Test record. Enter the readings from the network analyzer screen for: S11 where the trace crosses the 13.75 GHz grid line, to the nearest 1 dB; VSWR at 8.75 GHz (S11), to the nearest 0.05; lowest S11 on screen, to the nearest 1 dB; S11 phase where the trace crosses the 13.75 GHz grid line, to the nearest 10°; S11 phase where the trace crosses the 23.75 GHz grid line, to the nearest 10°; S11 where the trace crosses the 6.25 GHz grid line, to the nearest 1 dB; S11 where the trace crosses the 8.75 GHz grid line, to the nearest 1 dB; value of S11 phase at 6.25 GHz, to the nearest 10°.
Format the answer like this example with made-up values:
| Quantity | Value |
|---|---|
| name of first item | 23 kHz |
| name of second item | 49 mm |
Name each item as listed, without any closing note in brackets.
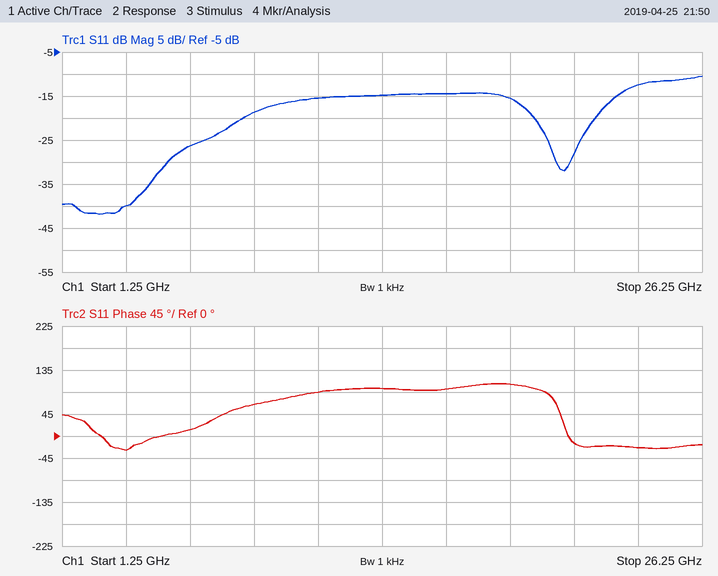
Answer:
| Quantity | Value |
|---|---|
| S11 where the trace crosses the 13.75 GHz grid line, to the nearest 1 dB | -15 dB |
| VSWR at 8.75 GHz (S11), to the nearest 0.05 | 1.25 |
| lowest S11 on screen, to the nearest 1 dB | -42 dB |
| S11 phase where the trace crosses the 13.75 GHz grid line, to the nearest 10° | 100° |
| S11 phase where the trace crosses the 23.75 GHz grid line, to the nearest 10° | -20° |
| S11 where the trace crosses the 6.25 GHz grid line, to the nearest 1 dB | -26 dB |
| S11 where the trace crosses the 8.75 GHz grid line, to the nearest 1 dB | -19 dB |
| value of S11 phase at 6.25 GHz, to the nearest 10° | 10° |
